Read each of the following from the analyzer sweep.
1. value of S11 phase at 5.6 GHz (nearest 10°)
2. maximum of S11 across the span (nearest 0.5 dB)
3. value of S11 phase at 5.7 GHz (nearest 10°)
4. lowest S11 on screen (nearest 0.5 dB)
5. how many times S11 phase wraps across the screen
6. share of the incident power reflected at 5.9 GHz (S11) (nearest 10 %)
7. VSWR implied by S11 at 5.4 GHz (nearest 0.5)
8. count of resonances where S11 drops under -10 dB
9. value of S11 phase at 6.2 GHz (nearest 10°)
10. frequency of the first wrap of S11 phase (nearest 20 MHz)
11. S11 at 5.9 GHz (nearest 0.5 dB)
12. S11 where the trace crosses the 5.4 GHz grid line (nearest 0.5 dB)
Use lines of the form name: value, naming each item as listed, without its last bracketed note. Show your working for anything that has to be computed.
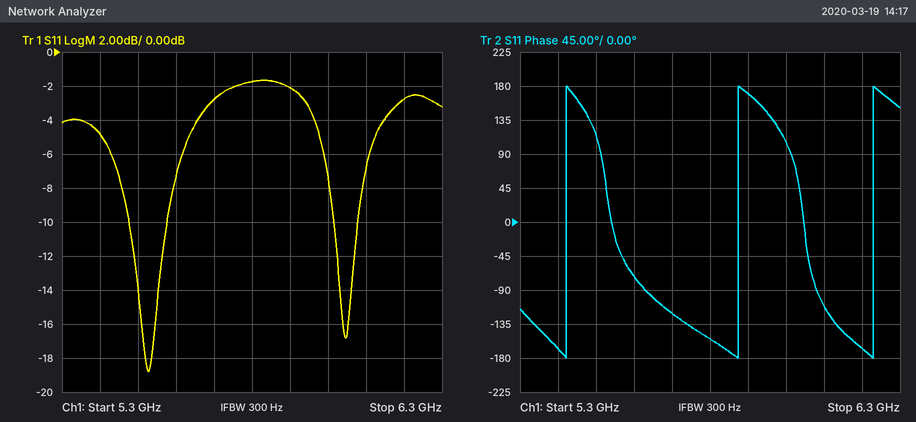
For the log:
value of S11 phase at 5.6 GHz: -70°
maximum of S11 across the span: -1.5 dB
value of S11 phase at 5.7 GHz: -120°
lowest S11 on screen: -19.0 dB
how many times S11 phase wraps across the screen: 3
share of the incident power reflected at 5.9 GHz (S11): 10^(-2/10) ≈ 63.1 %, so 60 % to the nearest 10 %
VSWR implied by S11 at 5.4 GHz: |Γ| = 10^(-5/20) = 0.5623; VSWR = (1 + 0.5623)/(1 − 0.5623) ≈ 3.57, so 3.5 to the nearest 0.5
count of resonances where S11 drops under -10 dB: 2
value of S11 phase at 6.2 GHz: -170°
frequency of the first wrap of S11 phase: 5.42 GHz
S11 at 5.9 GHz: -2.0 dB
S11 where the trace crosses the 5.4 GHz grid line: -5.0 dB
